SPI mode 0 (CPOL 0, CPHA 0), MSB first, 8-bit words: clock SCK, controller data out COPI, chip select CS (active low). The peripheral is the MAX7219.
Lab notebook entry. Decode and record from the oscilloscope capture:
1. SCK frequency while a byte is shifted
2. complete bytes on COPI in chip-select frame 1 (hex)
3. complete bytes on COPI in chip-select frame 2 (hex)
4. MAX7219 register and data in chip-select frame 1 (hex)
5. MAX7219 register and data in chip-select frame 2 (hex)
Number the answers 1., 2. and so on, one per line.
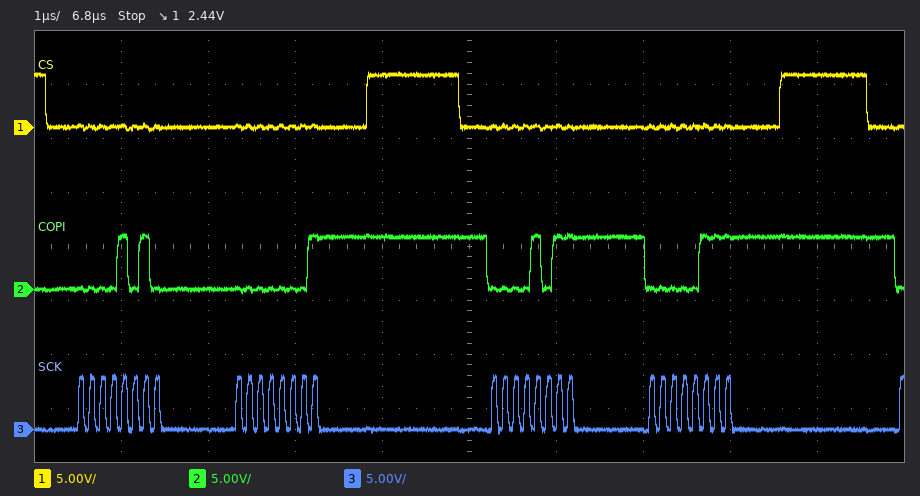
1. 8 MHz
2. 0A 01
3. 0B 07
4. register 0xA, data 0x01
5. register 0xB, data 0x07
